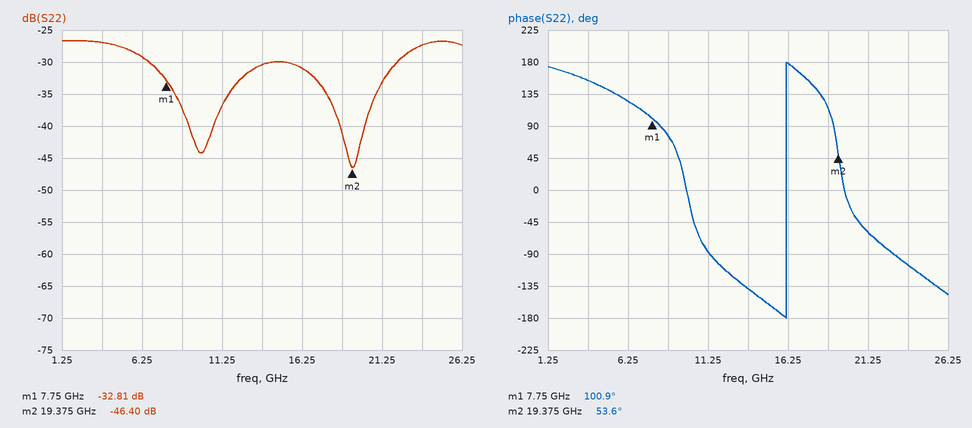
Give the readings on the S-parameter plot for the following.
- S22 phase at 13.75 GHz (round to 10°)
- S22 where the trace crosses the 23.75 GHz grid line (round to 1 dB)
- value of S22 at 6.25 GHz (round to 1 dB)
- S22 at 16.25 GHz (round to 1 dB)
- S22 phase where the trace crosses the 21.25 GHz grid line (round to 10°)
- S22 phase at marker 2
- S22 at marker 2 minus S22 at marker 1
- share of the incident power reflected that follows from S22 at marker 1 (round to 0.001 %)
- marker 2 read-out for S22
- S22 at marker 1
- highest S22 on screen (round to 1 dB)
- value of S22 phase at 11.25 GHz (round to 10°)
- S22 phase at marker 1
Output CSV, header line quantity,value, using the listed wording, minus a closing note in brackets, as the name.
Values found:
quantity,value
S22 phase at 13.75 GHz,-140°
S22 where the trace crosses the 23.75 GHz grid line,-27 dB
value of S22 at 6.25 GHz,-29 dB
S22 at 16.25 GHz,-31 dB
S22 phase where the trace crosses the 21.25 GHz grid line,-60°
S22 phase at marker 2,53.6°
S22 at marker 2 minus S22 at marker 1,-13.59 dB
share of the incident power reflected that follows from S22 at marker 1,0.052 %
marker 2 read-out for S22,-46.40 dB
S22 at marker 1,-32.81 dB
highest S22 on screen,-27 dB
value of S22 phase at 11.25 GHz,-90°
S22 phase at marker 1,100.9°
